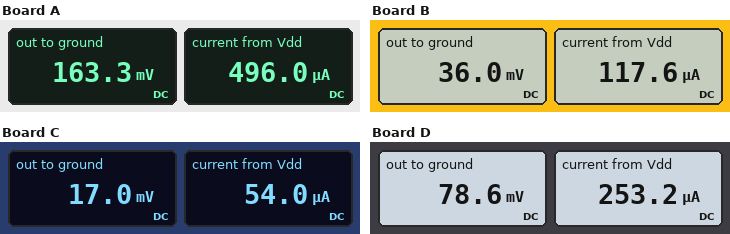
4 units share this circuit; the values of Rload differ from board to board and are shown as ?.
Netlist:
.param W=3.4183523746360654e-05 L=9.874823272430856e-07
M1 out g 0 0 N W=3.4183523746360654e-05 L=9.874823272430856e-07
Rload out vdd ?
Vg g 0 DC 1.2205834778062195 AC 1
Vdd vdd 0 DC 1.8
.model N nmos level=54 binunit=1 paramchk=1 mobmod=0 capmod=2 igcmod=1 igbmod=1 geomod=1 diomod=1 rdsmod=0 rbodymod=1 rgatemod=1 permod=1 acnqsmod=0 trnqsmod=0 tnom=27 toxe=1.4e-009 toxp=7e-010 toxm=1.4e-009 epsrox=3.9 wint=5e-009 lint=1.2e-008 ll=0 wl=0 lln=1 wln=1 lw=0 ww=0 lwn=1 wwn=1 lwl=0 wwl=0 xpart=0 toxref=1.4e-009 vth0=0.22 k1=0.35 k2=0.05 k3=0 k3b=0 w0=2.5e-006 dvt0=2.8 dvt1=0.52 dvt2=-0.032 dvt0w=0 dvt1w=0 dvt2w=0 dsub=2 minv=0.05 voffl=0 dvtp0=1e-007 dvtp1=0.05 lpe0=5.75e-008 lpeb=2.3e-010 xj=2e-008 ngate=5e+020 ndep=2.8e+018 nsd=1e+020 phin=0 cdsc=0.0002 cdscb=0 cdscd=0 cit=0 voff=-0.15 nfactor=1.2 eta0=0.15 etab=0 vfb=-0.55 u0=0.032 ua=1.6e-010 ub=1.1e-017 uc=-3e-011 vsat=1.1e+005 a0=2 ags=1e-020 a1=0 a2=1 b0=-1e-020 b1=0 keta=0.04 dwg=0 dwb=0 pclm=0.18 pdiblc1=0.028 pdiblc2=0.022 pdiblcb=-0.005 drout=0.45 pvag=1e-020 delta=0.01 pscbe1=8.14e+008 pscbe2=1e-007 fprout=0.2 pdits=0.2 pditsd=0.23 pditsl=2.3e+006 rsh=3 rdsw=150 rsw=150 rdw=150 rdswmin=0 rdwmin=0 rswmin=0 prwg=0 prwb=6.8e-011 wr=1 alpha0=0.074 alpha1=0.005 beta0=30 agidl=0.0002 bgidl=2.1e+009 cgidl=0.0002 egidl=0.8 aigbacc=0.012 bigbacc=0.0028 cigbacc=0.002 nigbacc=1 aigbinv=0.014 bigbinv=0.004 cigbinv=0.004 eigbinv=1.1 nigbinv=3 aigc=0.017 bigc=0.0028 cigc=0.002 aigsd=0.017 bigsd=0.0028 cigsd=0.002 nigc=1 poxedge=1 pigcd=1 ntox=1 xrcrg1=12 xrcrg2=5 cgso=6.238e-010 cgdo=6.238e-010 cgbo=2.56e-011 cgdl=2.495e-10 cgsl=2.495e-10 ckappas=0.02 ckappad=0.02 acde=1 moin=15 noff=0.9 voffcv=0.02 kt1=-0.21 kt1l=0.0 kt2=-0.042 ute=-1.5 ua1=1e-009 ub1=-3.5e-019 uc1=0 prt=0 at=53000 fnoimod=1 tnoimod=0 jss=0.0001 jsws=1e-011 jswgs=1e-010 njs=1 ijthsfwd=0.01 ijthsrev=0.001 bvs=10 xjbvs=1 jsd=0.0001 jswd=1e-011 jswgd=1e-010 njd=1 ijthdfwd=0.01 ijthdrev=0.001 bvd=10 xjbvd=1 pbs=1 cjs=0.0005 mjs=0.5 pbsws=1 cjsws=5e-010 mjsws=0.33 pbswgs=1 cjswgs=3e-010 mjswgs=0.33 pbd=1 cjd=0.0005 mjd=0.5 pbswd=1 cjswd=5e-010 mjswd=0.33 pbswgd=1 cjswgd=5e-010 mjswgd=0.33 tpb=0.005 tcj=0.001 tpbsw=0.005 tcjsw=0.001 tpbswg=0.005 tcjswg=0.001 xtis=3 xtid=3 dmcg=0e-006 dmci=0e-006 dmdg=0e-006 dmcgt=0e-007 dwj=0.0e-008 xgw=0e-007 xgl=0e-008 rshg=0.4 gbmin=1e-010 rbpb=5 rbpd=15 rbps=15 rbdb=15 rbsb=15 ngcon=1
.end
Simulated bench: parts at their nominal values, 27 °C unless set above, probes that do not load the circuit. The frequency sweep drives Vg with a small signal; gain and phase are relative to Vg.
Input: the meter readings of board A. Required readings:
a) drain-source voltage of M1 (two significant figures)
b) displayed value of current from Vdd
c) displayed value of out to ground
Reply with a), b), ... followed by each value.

a) 160 mV
b) 496.0 µA
c) 163.3 mV
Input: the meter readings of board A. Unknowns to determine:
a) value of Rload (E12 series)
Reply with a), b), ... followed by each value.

a) 3.3 kΩ
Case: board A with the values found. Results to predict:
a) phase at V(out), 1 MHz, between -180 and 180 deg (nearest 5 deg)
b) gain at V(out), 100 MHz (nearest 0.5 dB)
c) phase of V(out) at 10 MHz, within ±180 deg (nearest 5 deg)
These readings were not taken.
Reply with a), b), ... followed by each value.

a) 15 deg
b) -17.0 dB
c) 70 deg
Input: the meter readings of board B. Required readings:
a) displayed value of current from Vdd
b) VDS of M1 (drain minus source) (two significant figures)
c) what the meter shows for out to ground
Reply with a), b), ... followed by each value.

a) 117.6 µA
b) 36 mV
c) 36.0 mV
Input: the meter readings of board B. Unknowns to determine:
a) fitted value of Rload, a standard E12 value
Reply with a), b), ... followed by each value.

a) 15 kΩ
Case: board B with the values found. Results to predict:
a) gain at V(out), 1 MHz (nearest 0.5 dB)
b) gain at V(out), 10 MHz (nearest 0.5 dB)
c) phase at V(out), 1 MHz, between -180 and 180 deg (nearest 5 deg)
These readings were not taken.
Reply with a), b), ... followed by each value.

a) -41.0 dB
b) -36.0 dB
c) 10 deg
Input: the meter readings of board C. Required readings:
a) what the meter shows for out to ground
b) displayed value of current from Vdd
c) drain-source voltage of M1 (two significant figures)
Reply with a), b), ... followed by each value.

a) 17.0 mV
b) 54.0 µA
c) 17 mV
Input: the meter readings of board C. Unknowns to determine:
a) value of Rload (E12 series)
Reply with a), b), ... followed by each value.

a) 33 kΩ
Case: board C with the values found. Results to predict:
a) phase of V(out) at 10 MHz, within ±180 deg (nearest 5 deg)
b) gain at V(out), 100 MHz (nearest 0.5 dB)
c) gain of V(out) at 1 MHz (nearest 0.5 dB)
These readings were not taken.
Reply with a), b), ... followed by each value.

a) 60 deg
b) -18.0 dB
c) -42.5 dB
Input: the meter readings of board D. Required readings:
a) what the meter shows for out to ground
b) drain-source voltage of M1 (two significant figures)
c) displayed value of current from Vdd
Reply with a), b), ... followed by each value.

a) 78.6 mV
b) 79 mV
c) 253.2 µA
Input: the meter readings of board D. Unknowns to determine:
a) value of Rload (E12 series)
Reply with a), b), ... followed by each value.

a) 6.8 kΩ
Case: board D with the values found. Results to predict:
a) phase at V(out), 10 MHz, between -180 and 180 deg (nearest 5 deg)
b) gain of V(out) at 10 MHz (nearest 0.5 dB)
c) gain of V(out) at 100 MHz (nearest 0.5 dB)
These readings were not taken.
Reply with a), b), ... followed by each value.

a) 50 deg
b) -35.5 dB
c) -17.5 dB
